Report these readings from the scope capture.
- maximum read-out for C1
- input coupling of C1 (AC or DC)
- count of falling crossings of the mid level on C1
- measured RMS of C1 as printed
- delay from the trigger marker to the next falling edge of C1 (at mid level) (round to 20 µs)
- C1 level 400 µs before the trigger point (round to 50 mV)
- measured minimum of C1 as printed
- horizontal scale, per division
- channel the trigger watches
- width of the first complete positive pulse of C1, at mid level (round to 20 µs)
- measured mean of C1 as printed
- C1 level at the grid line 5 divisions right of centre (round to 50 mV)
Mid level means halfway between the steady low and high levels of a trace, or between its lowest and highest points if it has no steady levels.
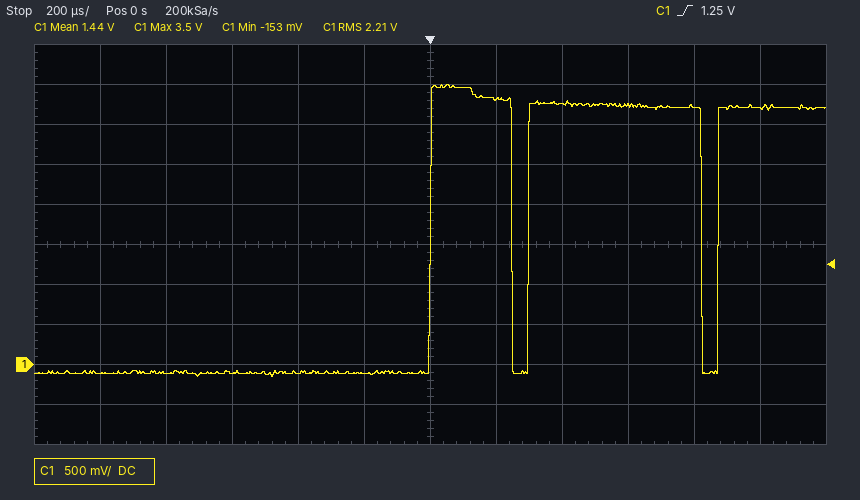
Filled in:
3.5 V
DC
2
2.21 V
240 µs
-100 mV
-153 mV
200 µs
C1
240 µs
1.44 V
3.20 V
